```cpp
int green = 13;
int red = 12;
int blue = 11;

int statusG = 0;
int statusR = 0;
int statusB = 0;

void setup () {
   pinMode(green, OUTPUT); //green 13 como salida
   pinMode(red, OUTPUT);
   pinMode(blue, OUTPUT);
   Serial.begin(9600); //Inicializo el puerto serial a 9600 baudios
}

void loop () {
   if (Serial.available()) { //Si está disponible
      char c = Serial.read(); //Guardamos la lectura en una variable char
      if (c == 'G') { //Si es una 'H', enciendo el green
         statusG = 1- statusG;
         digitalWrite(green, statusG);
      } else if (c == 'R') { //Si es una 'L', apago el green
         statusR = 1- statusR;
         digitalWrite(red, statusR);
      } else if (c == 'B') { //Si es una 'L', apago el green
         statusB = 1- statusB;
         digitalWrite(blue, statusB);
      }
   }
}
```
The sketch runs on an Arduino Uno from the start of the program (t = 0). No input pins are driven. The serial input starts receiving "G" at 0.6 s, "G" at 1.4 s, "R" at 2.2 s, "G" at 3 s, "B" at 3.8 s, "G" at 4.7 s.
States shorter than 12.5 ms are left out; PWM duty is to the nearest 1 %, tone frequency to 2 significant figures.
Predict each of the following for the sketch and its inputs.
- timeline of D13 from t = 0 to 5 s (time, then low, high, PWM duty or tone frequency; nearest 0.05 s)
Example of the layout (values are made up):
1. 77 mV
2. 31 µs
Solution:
1. 0 s low; 0.6 s high; 1.4 s low; 3 s high; 4.7 s low
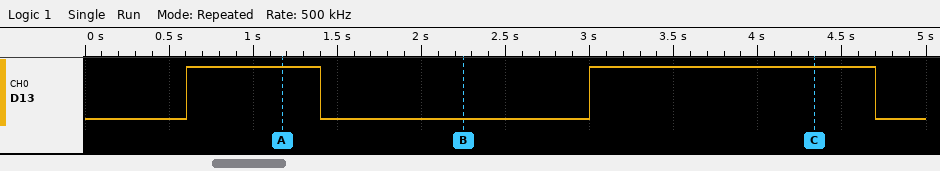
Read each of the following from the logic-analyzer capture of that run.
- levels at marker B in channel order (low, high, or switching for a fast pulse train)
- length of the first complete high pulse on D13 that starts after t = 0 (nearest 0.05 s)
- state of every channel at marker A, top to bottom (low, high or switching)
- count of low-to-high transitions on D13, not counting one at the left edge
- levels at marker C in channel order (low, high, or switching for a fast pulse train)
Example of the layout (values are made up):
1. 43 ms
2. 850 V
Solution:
1. D13 low
2. 0.80 s
3. D13 high
4. 2
5. D13 high
